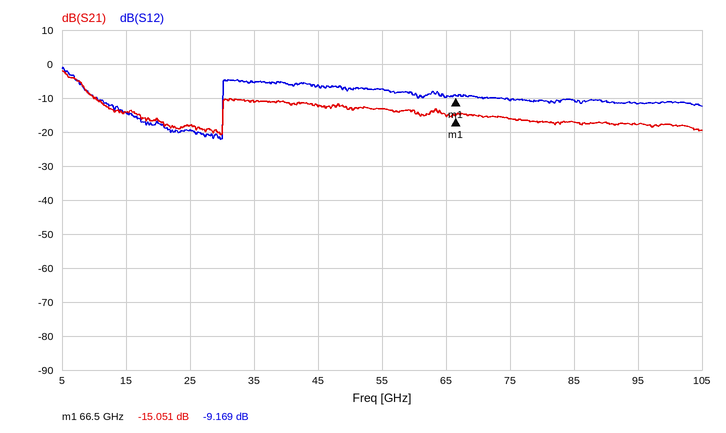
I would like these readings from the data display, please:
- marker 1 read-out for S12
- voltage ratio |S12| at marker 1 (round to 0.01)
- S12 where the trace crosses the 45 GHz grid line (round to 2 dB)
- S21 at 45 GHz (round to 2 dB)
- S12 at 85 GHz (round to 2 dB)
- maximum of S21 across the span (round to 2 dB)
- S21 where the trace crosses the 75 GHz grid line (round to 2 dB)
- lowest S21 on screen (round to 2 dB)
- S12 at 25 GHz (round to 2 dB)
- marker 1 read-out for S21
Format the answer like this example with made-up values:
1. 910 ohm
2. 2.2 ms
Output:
1. -9.169 dB
2. 0.35
3. -6 dB
4. -12 dB
5. -10 dB
6. -2 dB
7. -16 dB
8. -20 dB
9. -20 dB
10. -15.051 dB
